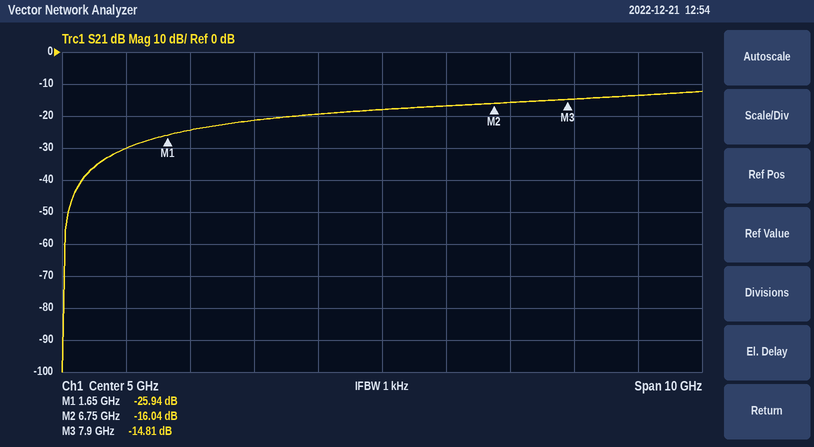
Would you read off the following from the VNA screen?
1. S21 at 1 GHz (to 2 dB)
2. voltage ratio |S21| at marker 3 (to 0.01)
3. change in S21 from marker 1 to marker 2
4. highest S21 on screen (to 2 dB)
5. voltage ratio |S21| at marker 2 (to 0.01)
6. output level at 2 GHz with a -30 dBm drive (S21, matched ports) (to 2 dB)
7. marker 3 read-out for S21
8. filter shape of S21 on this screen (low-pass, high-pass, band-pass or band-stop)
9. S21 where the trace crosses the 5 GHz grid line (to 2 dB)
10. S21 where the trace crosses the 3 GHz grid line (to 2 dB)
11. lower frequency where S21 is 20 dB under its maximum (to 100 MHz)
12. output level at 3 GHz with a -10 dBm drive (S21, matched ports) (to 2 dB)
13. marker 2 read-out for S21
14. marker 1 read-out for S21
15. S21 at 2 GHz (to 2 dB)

-30 dB
0.18
9.90 dB
-12 dB
0.16
-54 dBm
-14.81 dB
high-pass
-18 dB
-22 dB
800 MHz
-32 dBm
-16.04 dB
-25.94 dB
-24 dB
